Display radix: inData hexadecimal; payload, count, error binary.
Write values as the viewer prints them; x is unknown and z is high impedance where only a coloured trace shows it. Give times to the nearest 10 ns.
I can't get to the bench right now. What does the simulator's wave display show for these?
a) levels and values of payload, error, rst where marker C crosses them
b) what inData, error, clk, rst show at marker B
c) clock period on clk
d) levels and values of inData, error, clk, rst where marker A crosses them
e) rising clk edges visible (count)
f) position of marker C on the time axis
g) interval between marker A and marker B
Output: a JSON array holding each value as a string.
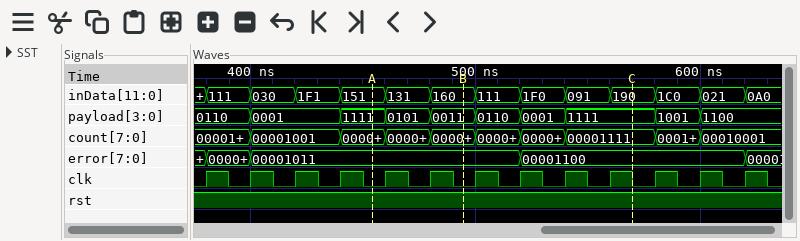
["payload=1111, error=00001100, rst=1", "inData=160, error=00001011, clk=0, rst=1", "20 ns", "inData=151, error=00001011, clk=0, rst=1", "13", "570 ns", "40 ns"]
